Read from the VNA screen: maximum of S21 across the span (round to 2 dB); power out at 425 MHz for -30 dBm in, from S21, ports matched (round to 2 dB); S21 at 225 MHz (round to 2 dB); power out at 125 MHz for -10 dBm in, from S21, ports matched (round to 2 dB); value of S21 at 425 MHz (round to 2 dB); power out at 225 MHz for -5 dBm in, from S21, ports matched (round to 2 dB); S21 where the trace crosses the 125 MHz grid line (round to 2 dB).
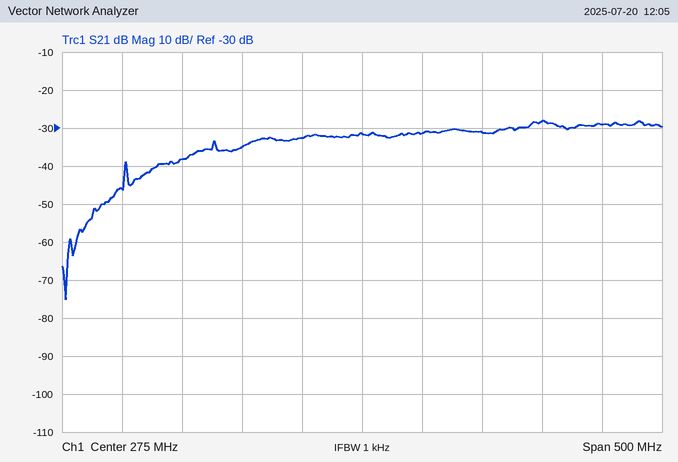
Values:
-28 dB
-58 dBm
-32 dB
-48 dBm
-28 dB
-38 dBm
-38 dB
